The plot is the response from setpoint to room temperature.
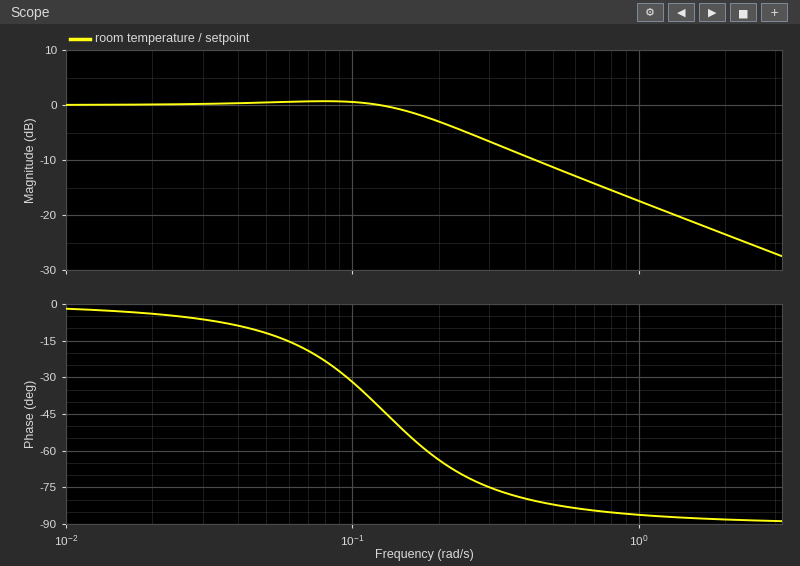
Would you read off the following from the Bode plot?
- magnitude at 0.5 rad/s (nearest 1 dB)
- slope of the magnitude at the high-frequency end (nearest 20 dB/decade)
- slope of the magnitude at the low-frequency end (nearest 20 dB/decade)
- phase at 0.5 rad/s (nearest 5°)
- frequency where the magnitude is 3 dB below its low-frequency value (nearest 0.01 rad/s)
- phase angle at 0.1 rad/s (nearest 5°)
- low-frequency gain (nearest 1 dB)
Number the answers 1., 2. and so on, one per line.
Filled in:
1. -11 dB
2. -20 dB/decade
3. 0 dB/decade
4. -80°
5. 0.20 rad/s
6. -30°
7. 0 dB
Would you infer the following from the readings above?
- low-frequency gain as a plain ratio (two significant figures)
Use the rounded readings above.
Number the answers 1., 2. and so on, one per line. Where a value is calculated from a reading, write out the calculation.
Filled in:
1. 10^(0 / 20) = 1.0
